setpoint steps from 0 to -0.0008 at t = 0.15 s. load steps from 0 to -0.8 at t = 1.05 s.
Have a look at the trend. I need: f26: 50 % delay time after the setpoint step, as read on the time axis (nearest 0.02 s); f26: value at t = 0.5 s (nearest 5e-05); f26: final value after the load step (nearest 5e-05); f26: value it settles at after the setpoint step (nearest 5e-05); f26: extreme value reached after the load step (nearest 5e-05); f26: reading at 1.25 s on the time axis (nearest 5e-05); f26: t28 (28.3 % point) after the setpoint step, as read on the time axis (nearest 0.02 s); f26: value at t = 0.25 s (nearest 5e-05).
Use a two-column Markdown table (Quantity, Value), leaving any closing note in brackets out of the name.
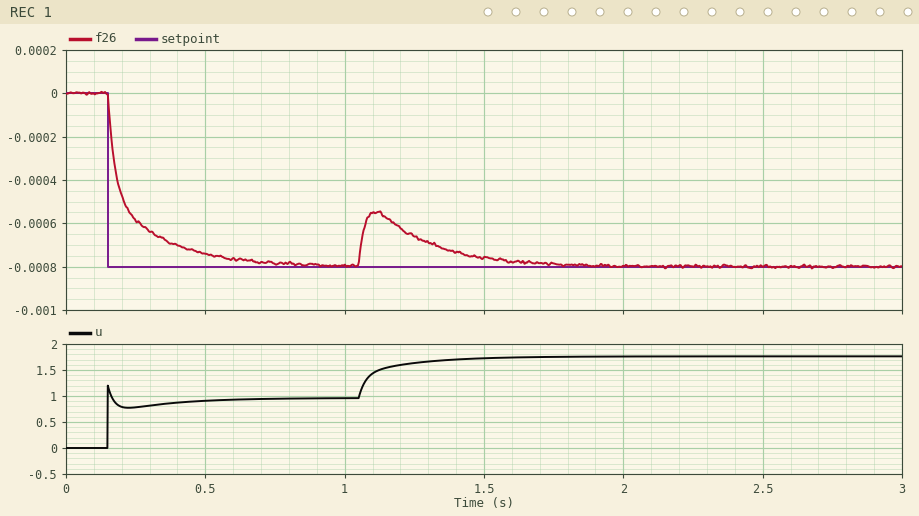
| Quantity | Value |
|---|---|
| f26: 50 % delay time after the setpoint step, as read on the time axis | 0.18 s |
| f26: value at t = 0.5 s | -0.00075 |
| f26: final value after the load step | -0.00080 |
| f26: value it settles at after the setpoint step | -0.00080 |
| f26: extreme value reached after the load step | -0.00055 |
| f26: reading at 1.25 s on the time axis | -0.00065 |
| f26: t28 (28.3 % point) after the setpoint step, as read on the time axis | 0.16 s |
| f26: value at t = 0.25 s | -0.00060 |
